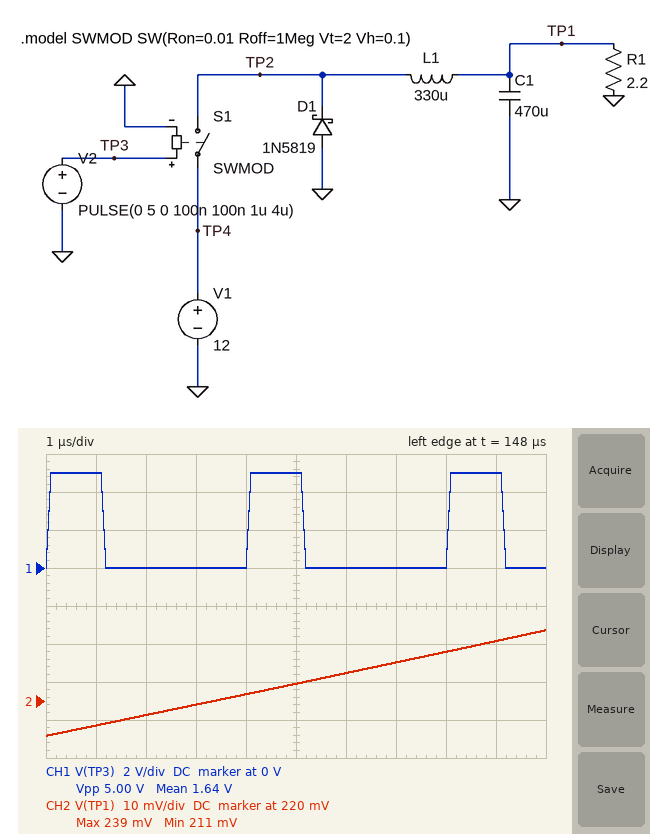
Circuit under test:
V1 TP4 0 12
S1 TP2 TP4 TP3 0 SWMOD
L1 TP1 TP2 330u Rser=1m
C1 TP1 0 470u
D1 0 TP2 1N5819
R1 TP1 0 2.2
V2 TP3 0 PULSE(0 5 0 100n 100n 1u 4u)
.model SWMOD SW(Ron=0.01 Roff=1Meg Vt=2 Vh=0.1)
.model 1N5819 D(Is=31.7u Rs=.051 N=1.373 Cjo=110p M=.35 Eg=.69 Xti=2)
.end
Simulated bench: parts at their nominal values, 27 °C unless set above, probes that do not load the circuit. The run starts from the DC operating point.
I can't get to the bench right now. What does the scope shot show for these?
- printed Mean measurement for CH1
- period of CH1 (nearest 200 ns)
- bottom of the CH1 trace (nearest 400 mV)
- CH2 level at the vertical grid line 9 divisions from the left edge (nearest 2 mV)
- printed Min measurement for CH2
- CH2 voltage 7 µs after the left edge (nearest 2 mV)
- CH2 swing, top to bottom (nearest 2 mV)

1.64 V
4.0 µs
0 V
236 mV
211 mV
230 mV
28 mV
